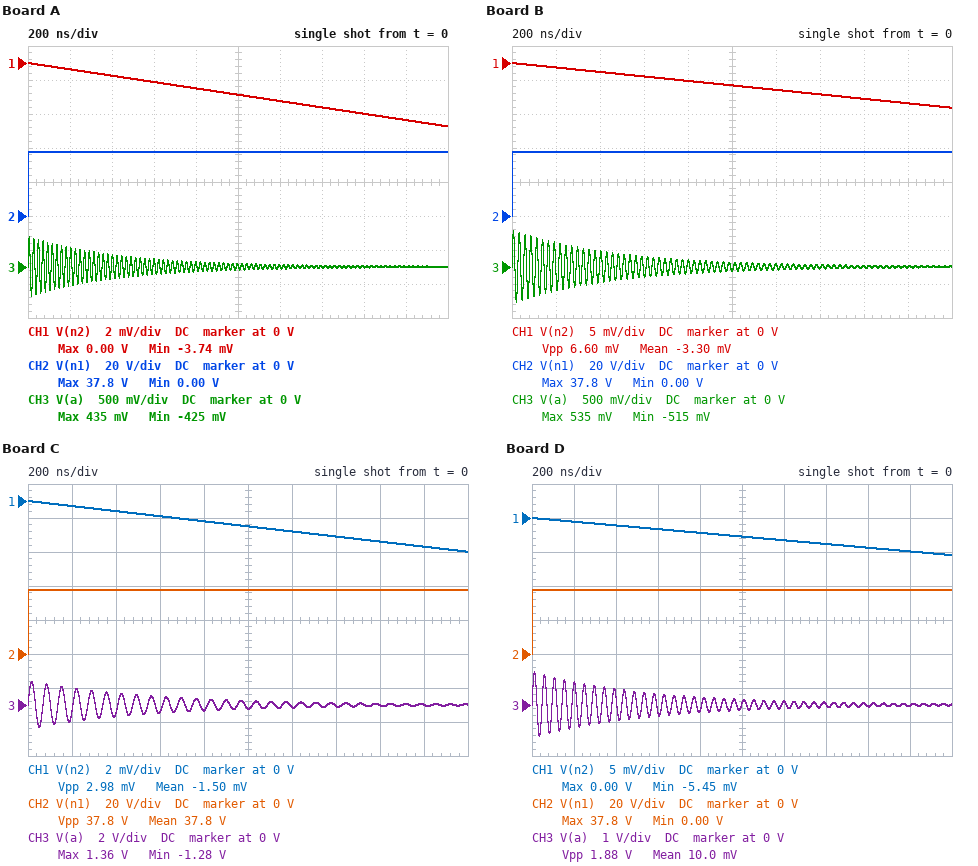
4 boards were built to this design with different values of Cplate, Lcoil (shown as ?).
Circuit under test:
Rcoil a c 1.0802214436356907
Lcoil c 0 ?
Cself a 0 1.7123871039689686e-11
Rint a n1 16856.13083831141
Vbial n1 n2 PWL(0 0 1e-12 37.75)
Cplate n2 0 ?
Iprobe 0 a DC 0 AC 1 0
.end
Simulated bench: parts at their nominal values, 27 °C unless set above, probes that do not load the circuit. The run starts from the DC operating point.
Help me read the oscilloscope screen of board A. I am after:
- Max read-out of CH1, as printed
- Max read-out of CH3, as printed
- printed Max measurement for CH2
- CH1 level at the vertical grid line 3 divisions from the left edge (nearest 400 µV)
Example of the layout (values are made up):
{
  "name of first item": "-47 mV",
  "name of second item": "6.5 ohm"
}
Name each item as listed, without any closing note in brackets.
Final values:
{
  "Max read-out of CH1, as printed": "0.00 V",
  "Max read-out of CH3, as printed": "435 mV",
  "printed Max measurement for CH2": "37.8 V",
  "CH1 level at the vertical grid line 3 divisions from the left edge": "-1.2 mV"
}
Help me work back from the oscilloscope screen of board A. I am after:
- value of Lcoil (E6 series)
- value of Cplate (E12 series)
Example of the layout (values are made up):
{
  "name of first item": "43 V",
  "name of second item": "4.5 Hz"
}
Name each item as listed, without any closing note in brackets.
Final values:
{
  "value of Lcoil": "680 nH",
  "value of Cplate": "1.2 µF"
}
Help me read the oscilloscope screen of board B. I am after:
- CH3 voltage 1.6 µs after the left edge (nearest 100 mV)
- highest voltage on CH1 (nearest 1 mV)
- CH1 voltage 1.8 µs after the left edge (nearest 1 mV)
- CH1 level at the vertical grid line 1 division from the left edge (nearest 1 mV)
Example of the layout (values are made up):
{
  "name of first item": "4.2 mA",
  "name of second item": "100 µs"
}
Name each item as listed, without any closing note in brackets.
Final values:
{
  "CH3 voltage 1.6 µs after the left edge": "0 V",
  "highest voltage on CH1": "0 V",
  "CH1 voltage 1.8 µs after the left edge": "-6 mV",
  "CH1 level at the vertical grid line 1 division from the left edge": "-1 mV"
}
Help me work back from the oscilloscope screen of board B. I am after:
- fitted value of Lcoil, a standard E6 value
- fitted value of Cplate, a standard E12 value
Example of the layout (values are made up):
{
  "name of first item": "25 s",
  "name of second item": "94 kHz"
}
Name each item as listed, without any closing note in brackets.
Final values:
{
  "fitted value of Lcoil, a standard E6 value": "1 µH",
  "fitted value of Cplate, a standard E12 value": "680 nF"
}
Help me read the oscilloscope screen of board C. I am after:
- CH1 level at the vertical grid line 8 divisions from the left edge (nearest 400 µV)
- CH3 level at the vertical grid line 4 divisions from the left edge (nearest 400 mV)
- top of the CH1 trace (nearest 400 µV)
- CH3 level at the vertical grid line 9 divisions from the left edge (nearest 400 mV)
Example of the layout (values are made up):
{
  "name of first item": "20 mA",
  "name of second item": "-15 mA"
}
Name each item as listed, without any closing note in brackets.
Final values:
{
  "CH1 level at the vertical grid line 8 divisions from the left edge": "-2.4 mV",
  "CH3 level at the vertical grid line 4 divisions from the left edge": "-400 mV",
  "top of the CH1 trace": "0 V",
  "CH3 level at the vertical grid line 9 divisions from the left edge": "0 V"
}
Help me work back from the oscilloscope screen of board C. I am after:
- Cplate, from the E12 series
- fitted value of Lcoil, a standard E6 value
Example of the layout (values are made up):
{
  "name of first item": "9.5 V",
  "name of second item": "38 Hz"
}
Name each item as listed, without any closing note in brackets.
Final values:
{
  "Cplate, from the E12 series": "1.5 µF",
  "fitted value of Lcoil, a standard E6 value": "6.8 µH"
}
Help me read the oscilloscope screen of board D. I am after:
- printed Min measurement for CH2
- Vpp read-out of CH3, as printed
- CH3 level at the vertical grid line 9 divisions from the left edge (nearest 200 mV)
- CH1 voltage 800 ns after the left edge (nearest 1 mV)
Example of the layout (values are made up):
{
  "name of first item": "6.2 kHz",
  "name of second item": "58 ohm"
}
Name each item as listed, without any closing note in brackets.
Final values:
{
  "printed Min measurement for CH2": "0.00 V",
  "Vpp read-out of CH3, as printed": "1.88 V",
  "CH3 level at the vertical grid line 9 divisions from the left edge": "0 V",
  "CH1 voltage 800 ns after the left edge": "-2 mV"
}
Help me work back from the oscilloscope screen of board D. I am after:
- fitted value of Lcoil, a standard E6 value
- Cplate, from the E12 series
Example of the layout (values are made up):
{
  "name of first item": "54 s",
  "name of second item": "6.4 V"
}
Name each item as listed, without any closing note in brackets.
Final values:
{
  "fitted value of Lcoil, a standard E6 value": "3.3 µH",
  "Cplate, from the E12 series": "820 nF"
}
